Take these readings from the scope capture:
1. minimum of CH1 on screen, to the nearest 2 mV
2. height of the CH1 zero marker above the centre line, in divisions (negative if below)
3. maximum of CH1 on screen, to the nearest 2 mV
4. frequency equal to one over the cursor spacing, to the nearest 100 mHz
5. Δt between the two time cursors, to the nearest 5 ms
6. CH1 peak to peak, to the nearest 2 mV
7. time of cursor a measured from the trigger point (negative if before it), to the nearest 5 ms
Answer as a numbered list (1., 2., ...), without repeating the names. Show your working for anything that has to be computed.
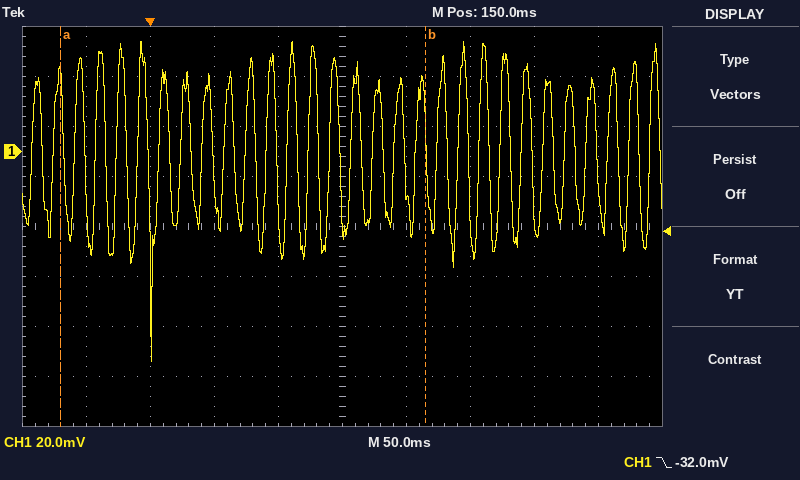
1. -84 mV
2. +1.5 div
3. 44 mV
4. 1 / 285 ms ≈ 3.5 Hz
5. 285 ms
6. 44 mV − (-84 mV) = 128 mV
7. -70 ms
